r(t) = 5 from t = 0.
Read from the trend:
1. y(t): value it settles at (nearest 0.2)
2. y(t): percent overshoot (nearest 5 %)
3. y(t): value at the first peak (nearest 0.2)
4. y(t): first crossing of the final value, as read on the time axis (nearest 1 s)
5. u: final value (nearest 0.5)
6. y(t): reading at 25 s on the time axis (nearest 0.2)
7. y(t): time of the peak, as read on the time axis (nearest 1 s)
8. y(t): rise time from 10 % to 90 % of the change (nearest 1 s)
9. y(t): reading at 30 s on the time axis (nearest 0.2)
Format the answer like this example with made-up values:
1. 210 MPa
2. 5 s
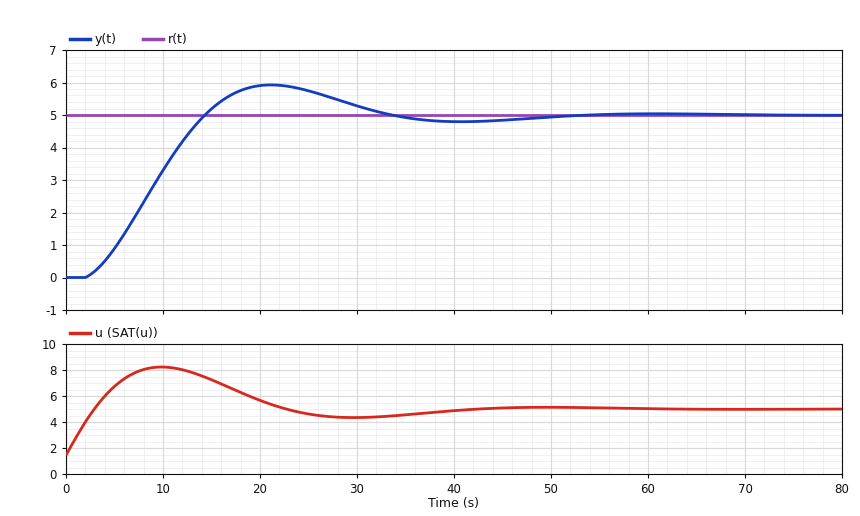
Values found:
1. 5.0
2. 20 %
3. 6.0
4. 14 s
5. 5.0
6. 5.8
7. 21 s
8. 9 s
9. 5.2
